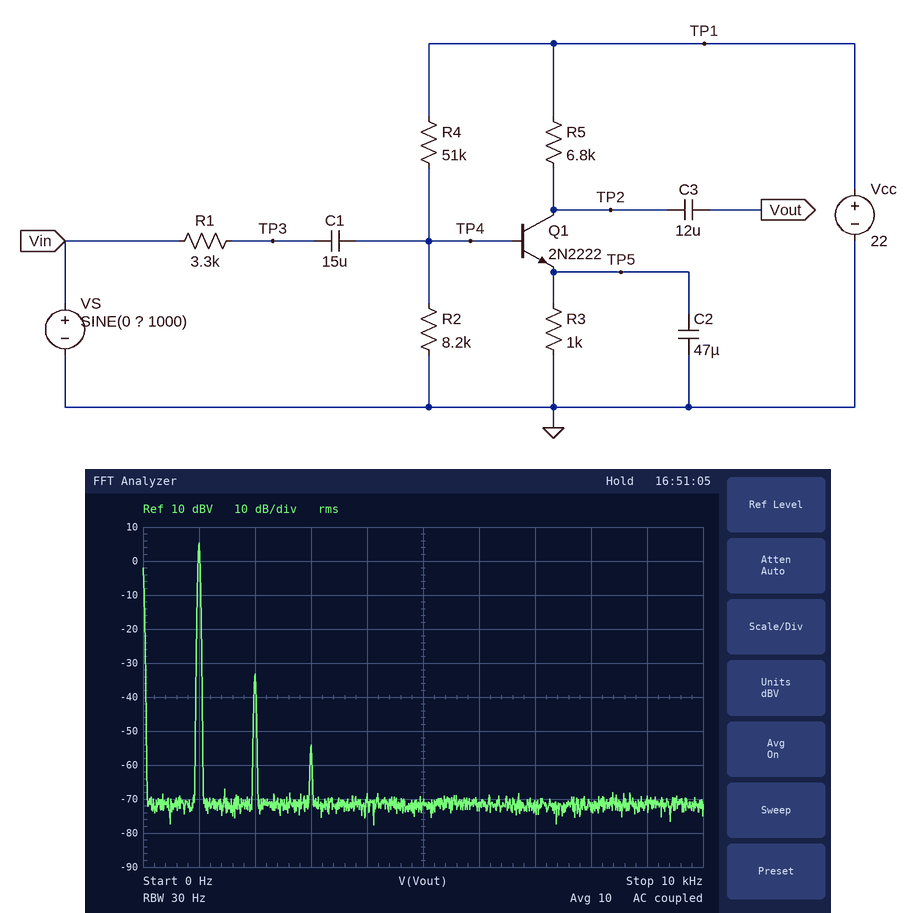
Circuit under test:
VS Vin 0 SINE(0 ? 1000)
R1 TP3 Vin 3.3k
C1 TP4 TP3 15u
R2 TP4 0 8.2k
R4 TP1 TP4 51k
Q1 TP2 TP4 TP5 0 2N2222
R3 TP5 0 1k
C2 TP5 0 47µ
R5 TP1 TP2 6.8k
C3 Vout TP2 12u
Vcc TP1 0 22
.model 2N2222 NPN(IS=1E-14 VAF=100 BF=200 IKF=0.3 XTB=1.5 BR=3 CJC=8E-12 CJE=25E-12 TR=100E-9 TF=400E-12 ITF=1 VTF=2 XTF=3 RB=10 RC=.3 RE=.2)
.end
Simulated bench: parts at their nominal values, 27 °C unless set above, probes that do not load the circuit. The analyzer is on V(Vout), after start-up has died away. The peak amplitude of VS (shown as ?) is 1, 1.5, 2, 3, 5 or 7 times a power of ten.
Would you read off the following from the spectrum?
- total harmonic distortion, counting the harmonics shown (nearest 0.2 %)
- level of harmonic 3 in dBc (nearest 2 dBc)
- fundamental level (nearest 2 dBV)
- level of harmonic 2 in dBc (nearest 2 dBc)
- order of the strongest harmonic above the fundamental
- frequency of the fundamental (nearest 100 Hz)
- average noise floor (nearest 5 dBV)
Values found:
1.2 %
-60 dBc
6 dBV
-38 dBc
2
1.0 kHz
-70 dBV
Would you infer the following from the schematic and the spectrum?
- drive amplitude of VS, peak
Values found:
15 mV
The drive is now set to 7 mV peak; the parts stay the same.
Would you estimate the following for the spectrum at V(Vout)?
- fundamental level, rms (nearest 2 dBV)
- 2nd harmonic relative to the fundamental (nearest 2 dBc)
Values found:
-2 dBV
-46 dBc
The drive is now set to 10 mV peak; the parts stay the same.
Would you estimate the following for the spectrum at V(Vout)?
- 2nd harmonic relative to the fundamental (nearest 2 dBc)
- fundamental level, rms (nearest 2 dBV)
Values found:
-42 dBc
2 dBV
